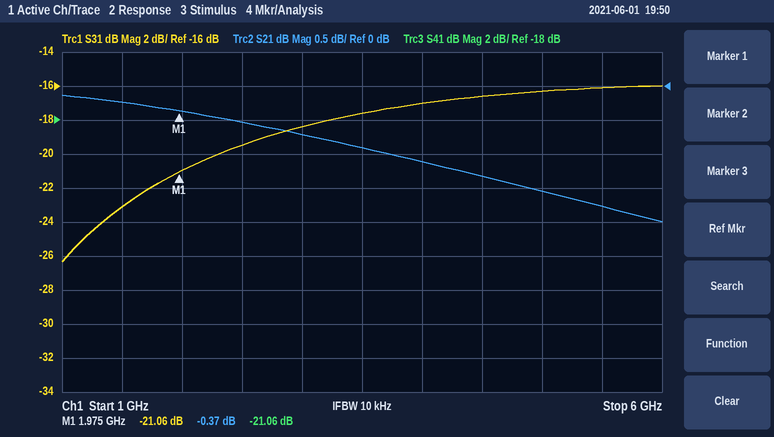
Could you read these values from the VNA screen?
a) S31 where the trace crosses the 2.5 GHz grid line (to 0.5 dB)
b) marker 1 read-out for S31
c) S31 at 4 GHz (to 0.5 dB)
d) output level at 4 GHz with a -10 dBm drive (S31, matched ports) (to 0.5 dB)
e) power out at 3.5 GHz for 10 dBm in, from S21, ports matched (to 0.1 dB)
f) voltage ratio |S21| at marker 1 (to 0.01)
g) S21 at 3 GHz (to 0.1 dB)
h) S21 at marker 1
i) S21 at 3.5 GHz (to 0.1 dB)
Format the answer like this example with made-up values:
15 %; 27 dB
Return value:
-19.5 dB; -21.06 dB; -17.0 dB; -27.0 dBm; 9.1 dBm; 0.96; -0.7 dB; -0.37 dB; -0.9 dB
